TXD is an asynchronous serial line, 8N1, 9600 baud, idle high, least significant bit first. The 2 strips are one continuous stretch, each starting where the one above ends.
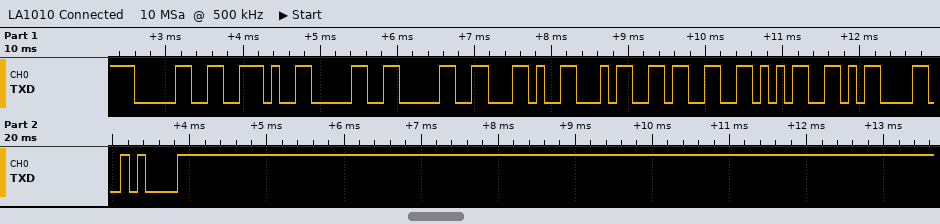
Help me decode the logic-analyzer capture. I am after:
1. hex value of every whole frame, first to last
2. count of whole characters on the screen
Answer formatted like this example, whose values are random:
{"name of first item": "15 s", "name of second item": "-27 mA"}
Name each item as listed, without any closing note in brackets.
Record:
{"hex value of every whole frame, first to last": "0x30 0x2E 0x30 0x30 0x2C 0x34 0x33 0x35 0x0D 0x0A", "count of whole characters on the screen": "10"}
